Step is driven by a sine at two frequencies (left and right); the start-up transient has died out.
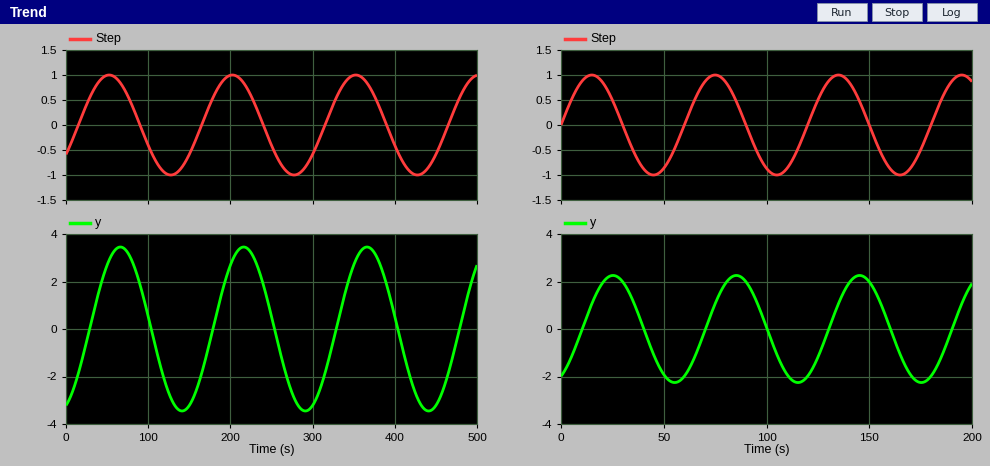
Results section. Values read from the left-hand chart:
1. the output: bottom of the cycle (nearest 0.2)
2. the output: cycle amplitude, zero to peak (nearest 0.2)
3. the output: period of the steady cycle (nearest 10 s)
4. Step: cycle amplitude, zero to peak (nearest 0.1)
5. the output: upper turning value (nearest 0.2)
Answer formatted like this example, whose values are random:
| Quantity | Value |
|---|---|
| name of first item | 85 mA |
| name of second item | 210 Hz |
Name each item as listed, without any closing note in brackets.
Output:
| Quantity | Value |
|---|---|
| the output: bottom of the cycle | -3.4 |
| the output: cycle amplitude, zero to peak | 3.4 |
| the output: period of the steady cycle | 150 s |
| Step: cycle amplitude, zero to peak | 1.0 |
| the output: upper turning value | 3.4 |
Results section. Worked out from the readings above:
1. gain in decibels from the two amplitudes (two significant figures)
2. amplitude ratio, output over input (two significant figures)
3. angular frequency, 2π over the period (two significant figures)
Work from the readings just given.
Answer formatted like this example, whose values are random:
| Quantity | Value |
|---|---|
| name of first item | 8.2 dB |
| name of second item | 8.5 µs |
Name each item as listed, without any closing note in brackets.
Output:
| Quantity | Value |
|---|---|
| gain in decibels from the two amplitudes | 11 dB |
| amplitude ratio, output over input | 3.4 |
| angular frequency, 2π over the period | 0.042 rad/s |
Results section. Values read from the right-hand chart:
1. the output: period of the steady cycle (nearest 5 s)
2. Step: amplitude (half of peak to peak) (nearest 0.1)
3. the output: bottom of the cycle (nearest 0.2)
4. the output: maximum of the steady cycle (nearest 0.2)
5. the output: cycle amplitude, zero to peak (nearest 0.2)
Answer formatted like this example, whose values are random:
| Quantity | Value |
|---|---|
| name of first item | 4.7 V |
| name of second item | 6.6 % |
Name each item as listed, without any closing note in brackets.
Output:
| Quantity | Value |
|---|---|
| the output: period of the steady cycle | 60 s |
| Step: amplitude (half of peak to peak) | 1.0 |
| the output: bottom of the cycle | -2.2 |
| the output: maximum of the steady cycle | 2.2 |
| the output: cycle amplitude, zero to peak | 2.2 |
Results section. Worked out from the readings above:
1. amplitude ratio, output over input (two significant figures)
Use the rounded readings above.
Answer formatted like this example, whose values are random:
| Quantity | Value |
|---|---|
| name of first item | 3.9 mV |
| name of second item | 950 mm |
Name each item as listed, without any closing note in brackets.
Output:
| Quantity | Value |
|---|---|
| amplitude ratio, output over input | 2.2 |
